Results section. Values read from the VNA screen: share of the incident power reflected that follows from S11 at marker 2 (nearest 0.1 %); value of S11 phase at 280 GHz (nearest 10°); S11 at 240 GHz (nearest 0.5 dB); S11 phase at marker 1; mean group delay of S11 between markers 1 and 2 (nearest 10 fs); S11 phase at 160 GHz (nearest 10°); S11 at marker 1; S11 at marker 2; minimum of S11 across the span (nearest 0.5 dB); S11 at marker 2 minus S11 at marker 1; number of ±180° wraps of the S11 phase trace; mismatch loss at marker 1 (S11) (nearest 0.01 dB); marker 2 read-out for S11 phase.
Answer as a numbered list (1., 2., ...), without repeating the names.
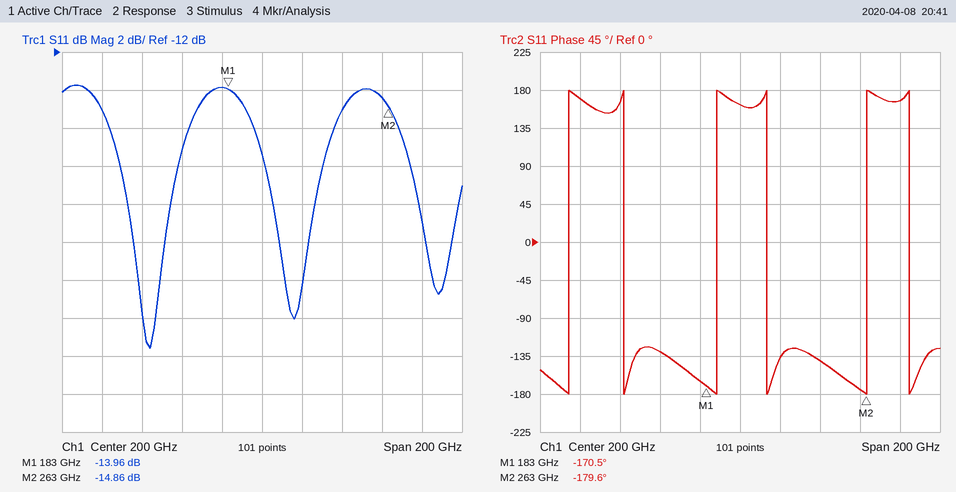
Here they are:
1. 3.3 %
2. 170°
3. -15.0 dB
4. -170.5°
5. 320 fs
6. -130°
7. -13.96 dB
8. -14.86 dB
9. -27.5 dB
10. -0.90 dB
11. 6
12. 0.18 dB
13. -179.6°
